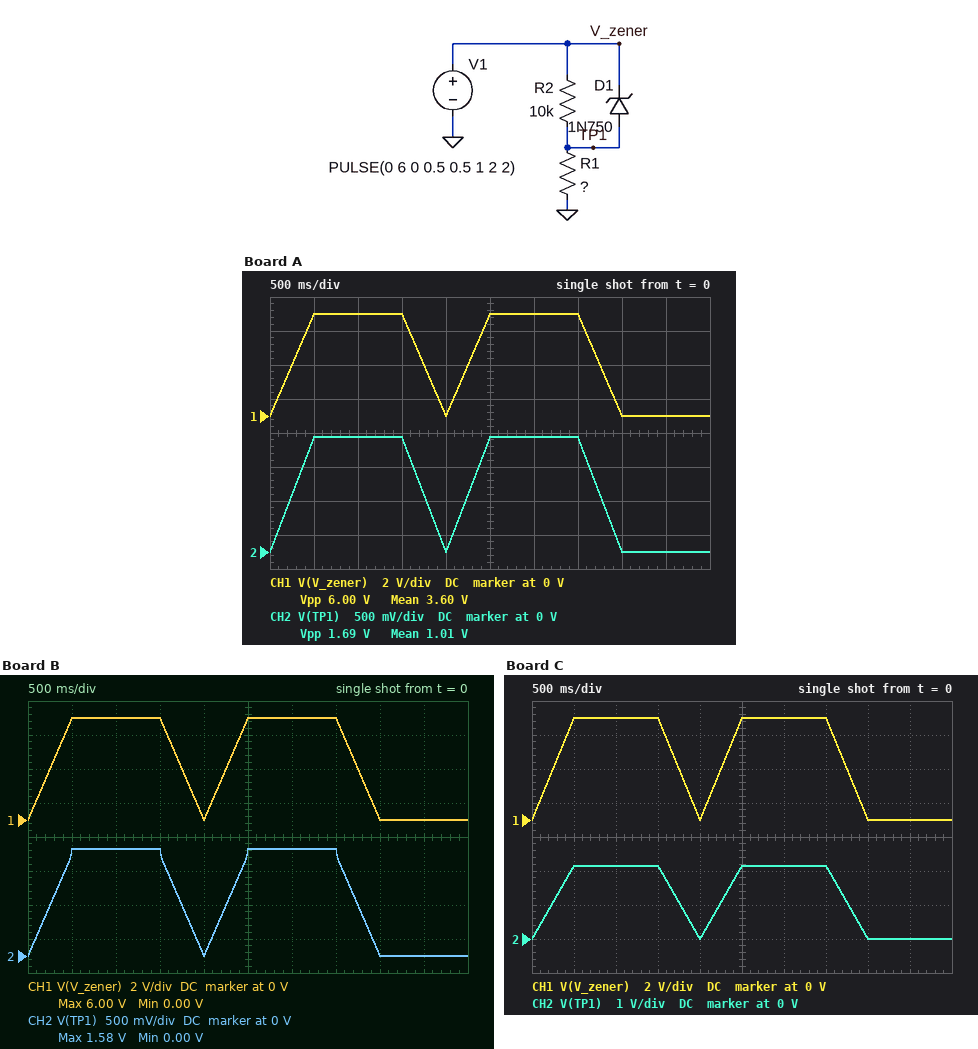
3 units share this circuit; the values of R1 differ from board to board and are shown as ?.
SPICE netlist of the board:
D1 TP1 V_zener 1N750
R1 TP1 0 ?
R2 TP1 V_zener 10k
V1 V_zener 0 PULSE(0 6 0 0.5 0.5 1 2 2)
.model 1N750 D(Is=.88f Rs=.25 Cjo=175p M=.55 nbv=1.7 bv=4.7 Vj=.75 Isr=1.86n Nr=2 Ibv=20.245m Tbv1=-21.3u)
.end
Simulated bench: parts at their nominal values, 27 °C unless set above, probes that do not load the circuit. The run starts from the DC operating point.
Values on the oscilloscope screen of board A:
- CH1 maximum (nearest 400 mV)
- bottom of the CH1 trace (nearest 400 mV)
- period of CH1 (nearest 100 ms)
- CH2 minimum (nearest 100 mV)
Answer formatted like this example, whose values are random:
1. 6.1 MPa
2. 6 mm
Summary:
1. 6.0 V
2. 0 V
3. 2.0 s
4. 0 V
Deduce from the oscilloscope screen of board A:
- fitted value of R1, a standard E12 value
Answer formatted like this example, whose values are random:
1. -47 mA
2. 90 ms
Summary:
1. 3.9 kΩ
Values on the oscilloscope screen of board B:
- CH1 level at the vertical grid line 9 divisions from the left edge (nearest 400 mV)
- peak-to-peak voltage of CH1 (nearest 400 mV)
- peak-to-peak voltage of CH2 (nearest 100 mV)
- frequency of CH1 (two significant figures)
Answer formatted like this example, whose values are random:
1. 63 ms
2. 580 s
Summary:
1. 0 V
2. 6.0 V
3. 1.6 V
4. 500 mHz
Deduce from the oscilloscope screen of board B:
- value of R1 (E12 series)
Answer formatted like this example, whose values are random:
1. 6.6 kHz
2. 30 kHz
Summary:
1. 3.3 kΩ
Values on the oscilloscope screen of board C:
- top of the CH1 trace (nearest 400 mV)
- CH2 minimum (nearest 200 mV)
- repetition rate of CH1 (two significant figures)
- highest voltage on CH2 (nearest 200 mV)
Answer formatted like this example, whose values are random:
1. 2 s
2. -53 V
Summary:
1. 6.0 V
2. 0 V
3. 500 mHz
4. 2.2 V
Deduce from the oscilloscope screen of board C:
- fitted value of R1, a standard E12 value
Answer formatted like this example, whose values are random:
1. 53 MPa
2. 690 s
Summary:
1. 5.6 kΩ
